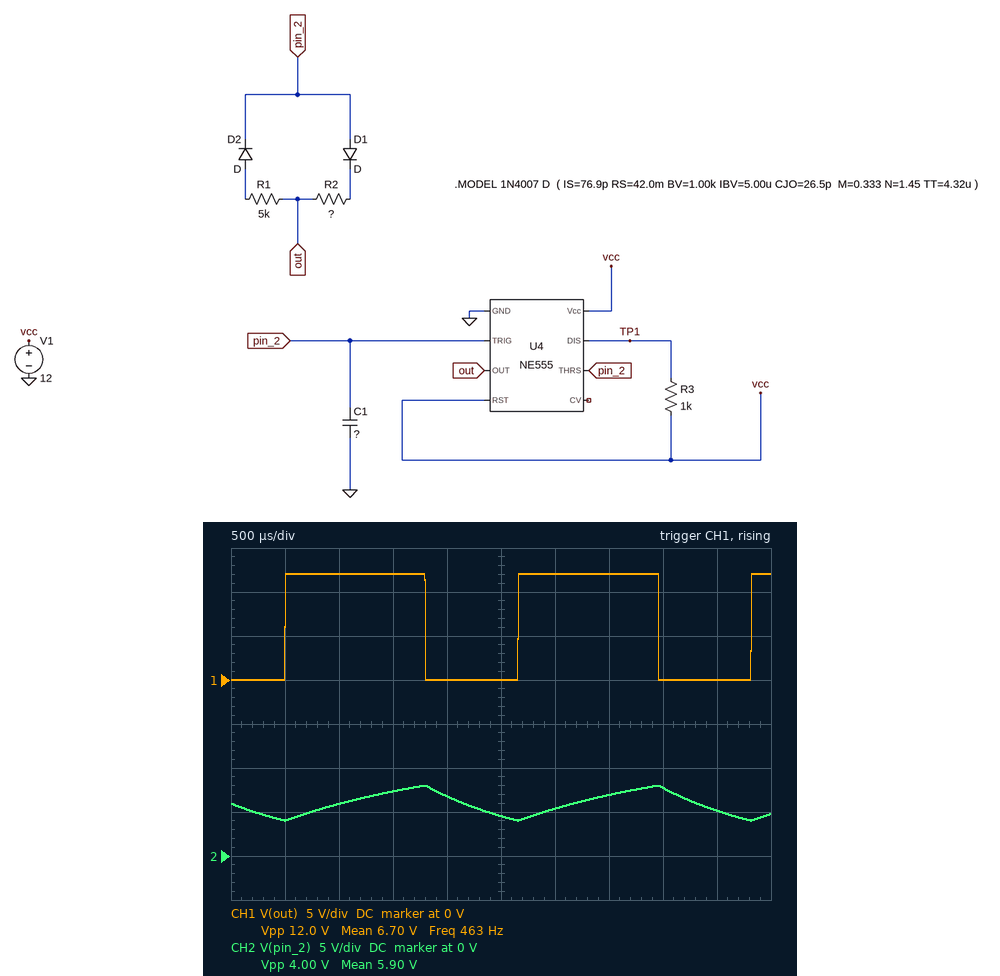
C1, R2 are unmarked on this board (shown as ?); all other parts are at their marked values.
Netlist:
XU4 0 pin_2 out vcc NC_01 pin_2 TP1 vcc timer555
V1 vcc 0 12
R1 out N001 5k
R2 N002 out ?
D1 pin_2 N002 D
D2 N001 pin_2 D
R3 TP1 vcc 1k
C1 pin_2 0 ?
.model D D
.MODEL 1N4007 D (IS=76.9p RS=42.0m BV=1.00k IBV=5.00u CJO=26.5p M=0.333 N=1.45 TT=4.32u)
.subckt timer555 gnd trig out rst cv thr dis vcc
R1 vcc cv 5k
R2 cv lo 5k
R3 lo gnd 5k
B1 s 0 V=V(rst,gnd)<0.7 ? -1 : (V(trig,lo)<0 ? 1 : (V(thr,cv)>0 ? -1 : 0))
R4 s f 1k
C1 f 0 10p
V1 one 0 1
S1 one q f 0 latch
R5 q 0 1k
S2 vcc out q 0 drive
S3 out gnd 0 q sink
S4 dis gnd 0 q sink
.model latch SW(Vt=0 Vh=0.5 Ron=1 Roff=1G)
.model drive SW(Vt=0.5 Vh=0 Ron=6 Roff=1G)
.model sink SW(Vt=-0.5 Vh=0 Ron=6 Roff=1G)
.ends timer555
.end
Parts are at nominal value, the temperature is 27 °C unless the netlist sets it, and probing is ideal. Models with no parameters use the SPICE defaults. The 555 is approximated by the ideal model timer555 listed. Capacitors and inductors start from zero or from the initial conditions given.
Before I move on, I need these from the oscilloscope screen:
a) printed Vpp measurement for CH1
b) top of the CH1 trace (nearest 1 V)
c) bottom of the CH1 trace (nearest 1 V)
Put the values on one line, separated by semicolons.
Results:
12.0 V; 12 V; 0 V
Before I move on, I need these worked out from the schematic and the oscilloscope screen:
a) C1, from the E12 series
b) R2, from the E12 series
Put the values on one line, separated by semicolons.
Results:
330 nF; 3.3 kΩ
